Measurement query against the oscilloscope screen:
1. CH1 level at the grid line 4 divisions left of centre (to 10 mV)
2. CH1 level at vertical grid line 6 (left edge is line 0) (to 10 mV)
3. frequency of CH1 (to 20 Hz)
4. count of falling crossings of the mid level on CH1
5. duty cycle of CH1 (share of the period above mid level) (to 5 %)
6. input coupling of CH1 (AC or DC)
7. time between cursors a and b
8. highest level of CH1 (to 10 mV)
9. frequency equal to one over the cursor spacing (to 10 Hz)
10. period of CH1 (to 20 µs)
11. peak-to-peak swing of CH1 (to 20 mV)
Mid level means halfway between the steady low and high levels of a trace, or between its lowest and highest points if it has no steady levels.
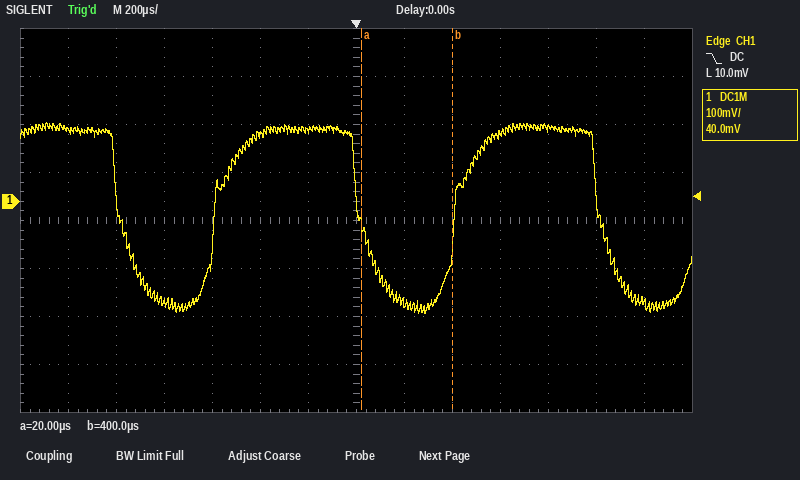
-210 mV
150 mV
1.00 kHz
3
60 %
DC
380 µs
160 mV
2.63 kHz
1.00 ms
400 mV
